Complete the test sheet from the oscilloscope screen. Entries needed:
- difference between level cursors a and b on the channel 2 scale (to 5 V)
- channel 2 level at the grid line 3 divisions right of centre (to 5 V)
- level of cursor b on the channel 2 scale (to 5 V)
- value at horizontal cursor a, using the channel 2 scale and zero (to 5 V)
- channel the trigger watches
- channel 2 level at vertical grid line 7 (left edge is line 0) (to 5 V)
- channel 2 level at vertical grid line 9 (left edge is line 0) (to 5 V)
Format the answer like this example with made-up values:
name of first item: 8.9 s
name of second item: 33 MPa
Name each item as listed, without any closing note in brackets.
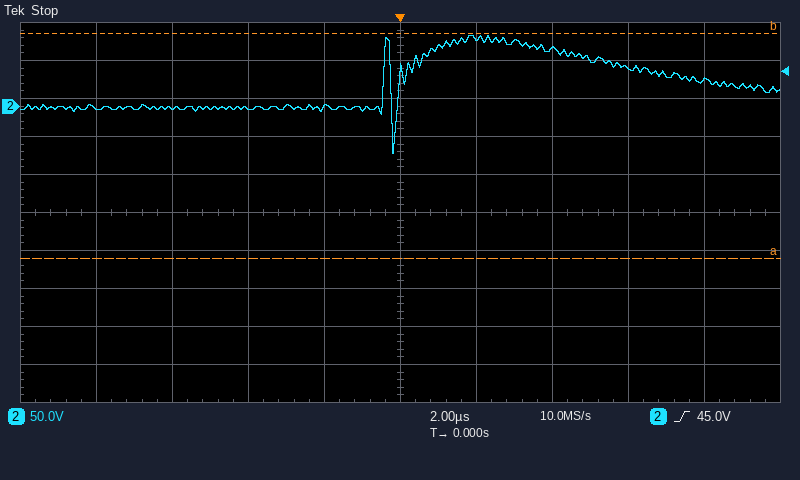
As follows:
difference between level cursors a and b on the channel 2 scale: 295 V
channel 2 level at the grid line 3 divisions right of centre: 50 V
level of cursor b on the channel 2 scale: 95 V
value at horizontal cursor a, using the channel 2 scale and zero: -200 V
channel the trigger watches: channel 2
channel 2 level at vertical grid line 7 (left edge is line 0): 75 V
channel 2 level at vertical grid line 9 (left edge is line 0): 35 V
